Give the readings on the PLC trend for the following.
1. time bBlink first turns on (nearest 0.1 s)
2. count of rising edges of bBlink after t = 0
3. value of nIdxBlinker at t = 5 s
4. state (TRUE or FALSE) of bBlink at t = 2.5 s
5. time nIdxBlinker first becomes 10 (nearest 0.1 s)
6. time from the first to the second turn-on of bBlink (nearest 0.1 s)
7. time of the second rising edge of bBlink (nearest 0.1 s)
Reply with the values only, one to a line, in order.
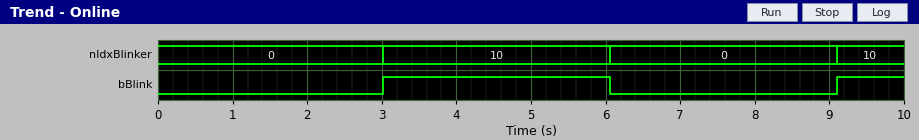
3.0 s
2
10
FALSE
3.0 s
6.1 s
9.1 s
